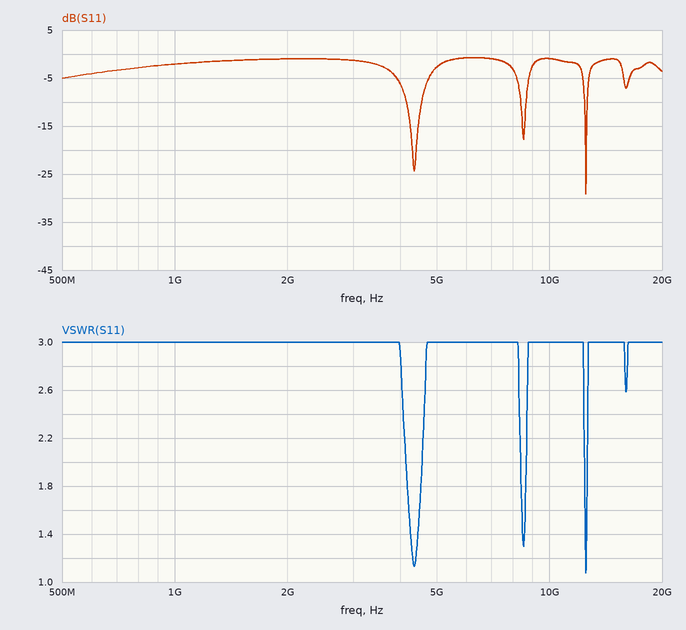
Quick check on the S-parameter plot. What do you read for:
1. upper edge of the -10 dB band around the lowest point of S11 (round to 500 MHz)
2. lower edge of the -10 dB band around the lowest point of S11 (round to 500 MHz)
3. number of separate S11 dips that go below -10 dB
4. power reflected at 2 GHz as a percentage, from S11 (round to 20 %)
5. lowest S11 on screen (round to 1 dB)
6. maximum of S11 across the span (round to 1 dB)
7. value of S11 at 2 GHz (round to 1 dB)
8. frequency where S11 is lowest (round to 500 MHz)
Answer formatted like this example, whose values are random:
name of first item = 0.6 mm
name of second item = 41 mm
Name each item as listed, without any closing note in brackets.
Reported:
upper edge of the -10 dB band around the lowest point of S11 = 12.5 GHz
lower edge of the -10 dB band around the lowest point of S11 = 12.5 GHz
number of separate S11 dips that go below -10 dB = 3
power reflected at 2 GHz as a percentage, from S11 = 80 %
lowest S11 on screen = -29 dB
maximum of S11 across the span = -1 dB
value of S11 at 2 GHz = -1 dB
frequency where S11 is lowest = 12.5 GHz
